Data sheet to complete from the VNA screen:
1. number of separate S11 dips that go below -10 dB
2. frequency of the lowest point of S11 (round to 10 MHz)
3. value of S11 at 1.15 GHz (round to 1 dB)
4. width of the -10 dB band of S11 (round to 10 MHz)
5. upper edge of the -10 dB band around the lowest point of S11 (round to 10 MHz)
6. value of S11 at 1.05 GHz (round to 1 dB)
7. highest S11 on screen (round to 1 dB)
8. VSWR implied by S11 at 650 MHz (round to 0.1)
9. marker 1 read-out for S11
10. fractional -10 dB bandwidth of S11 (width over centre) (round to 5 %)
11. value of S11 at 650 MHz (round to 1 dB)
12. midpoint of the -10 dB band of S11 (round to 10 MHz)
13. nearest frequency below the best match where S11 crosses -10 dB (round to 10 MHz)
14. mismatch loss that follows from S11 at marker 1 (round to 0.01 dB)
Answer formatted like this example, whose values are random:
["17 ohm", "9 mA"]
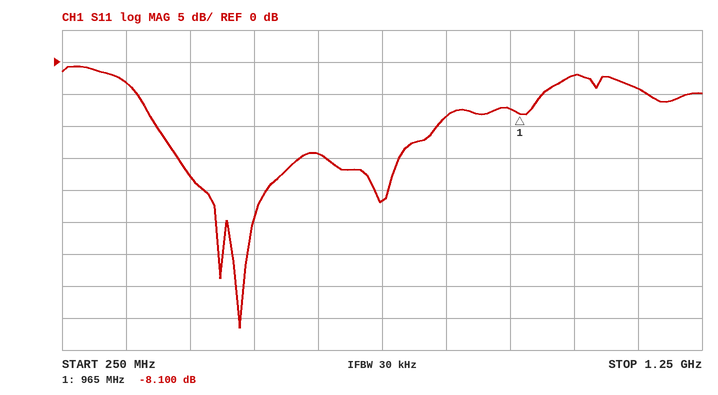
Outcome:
["3", "530 MHz", "-4 dB", "440 MHz", "840 MHz", "-2 dB", "-1 dB", "1.5", "-8.100 dB", "70 %", "-14 dB", "620 MHz", "400 MHz", "0.73 dB"]
